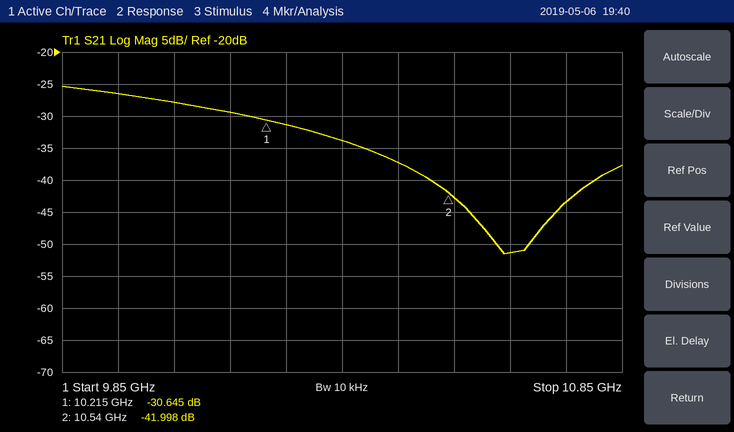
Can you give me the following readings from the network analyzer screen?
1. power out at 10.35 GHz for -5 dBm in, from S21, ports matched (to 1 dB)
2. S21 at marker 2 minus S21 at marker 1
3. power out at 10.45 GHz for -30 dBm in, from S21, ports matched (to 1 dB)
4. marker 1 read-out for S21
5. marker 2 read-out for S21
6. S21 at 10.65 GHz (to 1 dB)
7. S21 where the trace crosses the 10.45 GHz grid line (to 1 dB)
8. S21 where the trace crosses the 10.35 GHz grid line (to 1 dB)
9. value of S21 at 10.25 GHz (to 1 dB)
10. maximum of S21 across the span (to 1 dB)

-39 dBm
-11.353 dB
-67 dBm
-30.645 dB
-41.998 dB
-51 dB
-37 dB
-34 dB
-31 dB
-25 dB
